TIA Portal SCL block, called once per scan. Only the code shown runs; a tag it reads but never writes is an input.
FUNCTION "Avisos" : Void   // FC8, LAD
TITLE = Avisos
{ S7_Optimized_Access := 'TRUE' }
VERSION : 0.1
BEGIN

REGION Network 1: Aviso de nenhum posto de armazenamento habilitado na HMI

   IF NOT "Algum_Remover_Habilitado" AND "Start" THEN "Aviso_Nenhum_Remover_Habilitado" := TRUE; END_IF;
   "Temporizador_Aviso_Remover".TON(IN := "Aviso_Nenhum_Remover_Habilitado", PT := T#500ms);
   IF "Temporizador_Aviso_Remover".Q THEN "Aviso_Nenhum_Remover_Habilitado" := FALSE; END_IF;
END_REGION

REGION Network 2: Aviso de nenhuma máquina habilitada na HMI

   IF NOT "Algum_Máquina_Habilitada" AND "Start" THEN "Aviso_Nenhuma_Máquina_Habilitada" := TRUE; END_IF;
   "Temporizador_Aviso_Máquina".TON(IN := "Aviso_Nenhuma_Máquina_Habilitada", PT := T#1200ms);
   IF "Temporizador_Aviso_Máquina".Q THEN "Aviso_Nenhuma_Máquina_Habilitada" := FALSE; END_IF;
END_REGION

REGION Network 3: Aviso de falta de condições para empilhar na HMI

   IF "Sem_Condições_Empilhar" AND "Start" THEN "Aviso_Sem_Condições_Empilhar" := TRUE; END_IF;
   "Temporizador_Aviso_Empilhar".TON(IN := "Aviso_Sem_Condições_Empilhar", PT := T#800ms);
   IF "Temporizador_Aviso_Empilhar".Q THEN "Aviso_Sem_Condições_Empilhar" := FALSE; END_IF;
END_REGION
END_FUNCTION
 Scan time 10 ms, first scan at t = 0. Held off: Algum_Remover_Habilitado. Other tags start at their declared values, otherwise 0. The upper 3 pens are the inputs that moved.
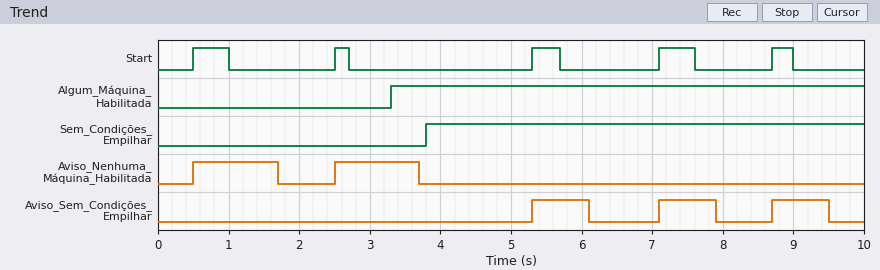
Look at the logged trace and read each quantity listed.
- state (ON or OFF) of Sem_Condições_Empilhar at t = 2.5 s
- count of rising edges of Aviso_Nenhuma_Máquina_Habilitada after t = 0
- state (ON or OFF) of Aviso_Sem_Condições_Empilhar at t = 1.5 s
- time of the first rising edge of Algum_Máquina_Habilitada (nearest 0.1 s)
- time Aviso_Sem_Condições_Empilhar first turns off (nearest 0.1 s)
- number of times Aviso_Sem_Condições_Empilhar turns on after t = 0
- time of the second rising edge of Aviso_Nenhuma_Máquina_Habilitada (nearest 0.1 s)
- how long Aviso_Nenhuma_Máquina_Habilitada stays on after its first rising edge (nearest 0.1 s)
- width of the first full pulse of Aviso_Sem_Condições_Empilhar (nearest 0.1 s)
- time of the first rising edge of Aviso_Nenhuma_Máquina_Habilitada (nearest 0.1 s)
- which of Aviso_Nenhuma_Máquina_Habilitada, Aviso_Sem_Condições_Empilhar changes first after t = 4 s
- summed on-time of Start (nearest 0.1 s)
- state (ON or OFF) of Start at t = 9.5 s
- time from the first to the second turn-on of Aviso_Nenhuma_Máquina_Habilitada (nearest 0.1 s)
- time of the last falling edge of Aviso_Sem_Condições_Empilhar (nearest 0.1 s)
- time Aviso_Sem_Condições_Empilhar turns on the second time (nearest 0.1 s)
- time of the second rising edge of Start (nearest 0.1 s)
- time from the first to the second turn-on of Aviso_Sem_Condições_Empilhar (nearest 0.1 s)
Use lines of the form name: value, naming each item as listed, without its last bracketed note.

state (ON or OFF) of Sem_Condições_Empilhar at t = 2.5 s: OFF
count of rising edges of Aviso_Nenhuma_Máquina_Habilitada after t = 0: 2
state (ON or OFF) of Aviso_Sem_Condições_Empilhar at t = 1.5 s: OFF
time of the first rising edge of Algum_Máquina_Habilitada: 3.3 s
time Aviso_Sem_Condições_Empilhar first turns off: 6.1 s
number of times Aviso_Sem_Condições_Empilhar turns on after t = 0: 3
time of the second rising edge of Aviso_Nenhuma_Máquina_Habilitada: 2.5 s
how long Aviso_Nenhuma_Máquina_Habilitada stays on after its first rising edge: 1.2 s
width of the first full pulse of Aviso_Sem_Condições_Empilhar: 0.8 s
time of the first rising edge of Aviso_Nenhuma_Máquina_Habilitada: 0.5 s
which of Aviso_Nenhuma_Máquina_Habilitada, Aviso_Sem_Condições_Empilhar changes first after t = 4 s: Aviso_Sem_Condições_Empilhar
summed on-time of Start: 1.9 s
state (ON or OFF) of Start at t = 9.5 s: OFF
time from the first to the second turn-on of Aviso_Nenhuma_Máquina_Habilitada: 2.0 s
time of the last falling edge of Aviso_Sem_Condições_Empilhar: 9.5 s
time Aviso_Sem_Condições_Empilhar turns on the second time: 7.1 s
time of the second rising edge of Start: 2.5 s
time from the first to the second turn-on of Aviso_Sem_Condições_Empilhar: 1.8 s
